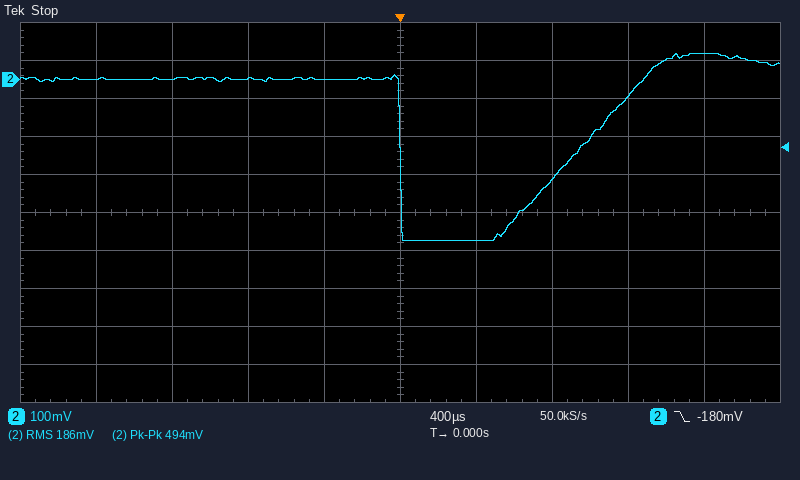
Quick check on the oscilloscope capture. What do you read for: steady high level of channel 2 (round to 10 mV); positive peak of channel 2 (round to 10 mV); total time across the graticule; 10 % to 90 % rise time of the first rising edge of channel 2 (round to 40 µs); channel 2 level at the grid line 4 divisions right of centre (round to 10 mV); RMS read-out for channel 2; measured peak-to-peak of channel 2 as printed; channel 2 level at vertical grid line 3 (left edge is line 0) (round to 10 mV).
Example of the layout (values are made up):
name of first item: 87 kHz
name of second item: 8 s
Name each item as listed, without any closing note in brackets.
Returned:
steady high level of channel 2: 0 mV
positive peak of channel 2: 70 mV
total time across the graticule: 4 ms
10 % to 90 % rise time of the first rising edge of channel 2: 640 µs
channel 2 level at the grid line 4 divisions right of centre: 70 mV
RMS read-out for channel 2: 186 mV
measured peak-to-peak of channel 2 as printed: 494 mV
channel 2 level at vertical grid line 3 (left edge is line 0): 0 mV
